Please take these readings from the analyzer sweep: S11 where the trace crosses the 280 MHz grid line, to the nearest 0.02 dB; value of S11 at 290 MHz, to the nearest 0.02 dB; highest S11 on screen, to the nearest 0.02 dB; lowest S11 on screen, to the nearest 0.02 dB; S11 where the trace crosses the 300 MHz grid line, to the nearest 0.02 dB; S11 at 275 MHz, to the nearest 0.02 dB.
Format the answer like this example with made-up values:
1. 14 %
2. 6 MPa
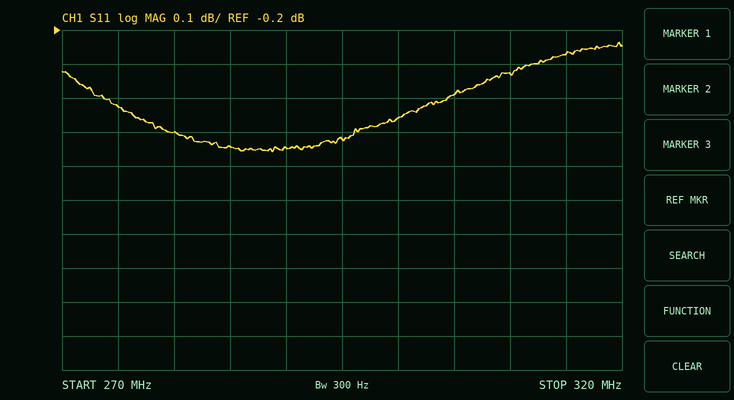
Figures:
1. -0.50 dB
2. -0.54 dB
3. -0.24 dB
4. -0.56 dB
5. -0.46 dB
6. -0.42 dB
